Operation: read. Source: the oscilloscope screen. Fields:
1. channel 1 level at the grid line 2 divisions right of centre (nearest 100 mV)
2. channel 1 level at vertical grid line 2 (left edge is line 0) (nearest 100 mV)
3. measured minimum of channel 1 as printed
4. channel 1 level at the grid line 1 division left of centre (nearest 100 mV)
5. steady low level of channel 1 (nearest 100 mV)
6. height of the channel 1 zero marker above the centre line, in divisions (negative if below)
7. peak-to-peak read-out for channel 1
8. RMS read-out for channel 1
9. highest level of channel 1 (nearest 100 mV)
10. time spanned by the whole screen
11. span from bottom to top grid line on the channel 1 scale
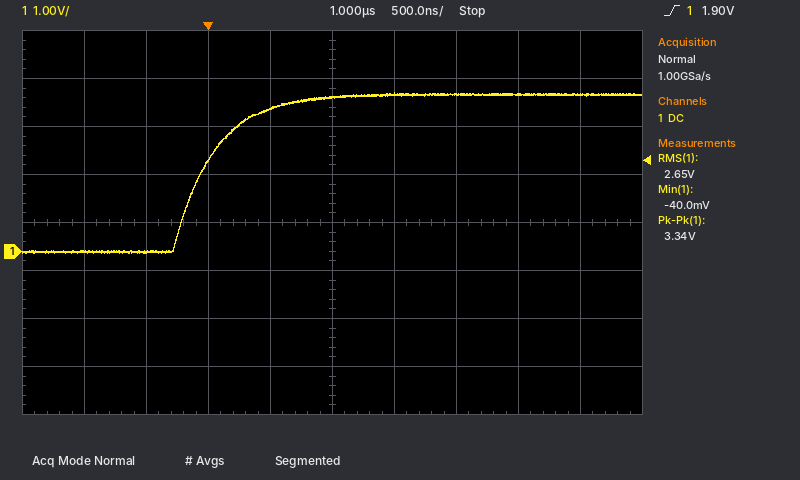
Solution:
3.3 V
0.0 V
-40.0 mV
3.0 V
0.0 V
-0.6 div
3.34 V
2.65 V
3.3 V
5 µs
8 V
